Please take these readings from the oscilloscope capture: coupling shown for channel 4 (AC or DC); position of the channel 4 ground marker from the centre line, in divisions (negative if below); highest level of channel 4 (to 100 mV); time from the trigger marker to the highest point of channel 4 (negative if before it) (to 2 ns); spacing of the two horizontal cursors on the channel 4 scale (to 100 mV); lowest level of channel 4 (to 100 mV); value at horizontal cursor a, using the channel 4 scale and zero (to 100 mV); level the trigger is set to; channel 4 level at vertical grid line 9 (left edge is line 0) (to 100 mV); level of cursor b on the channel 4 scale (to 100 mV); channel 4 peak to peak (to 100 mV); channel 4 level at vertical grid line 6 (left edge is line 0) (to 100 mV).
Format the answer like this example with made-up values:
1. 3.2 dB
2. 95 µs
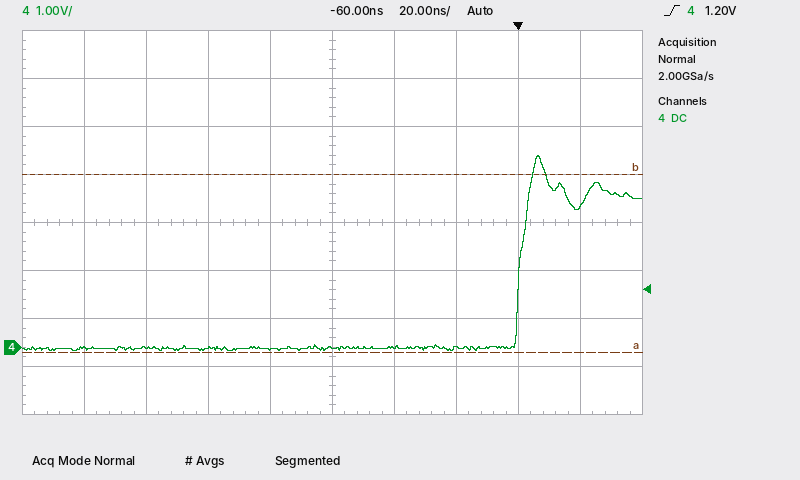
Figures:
1. DC
2. -2.6 div
3. 4.0 V
4. +6 ns
5. 3.7 V
6. -100 mV
7. -100 mV
8. 1.20 V
9. 2.9 V
10. 3.6 V
11. 4.1 V
12. 0.0 V
